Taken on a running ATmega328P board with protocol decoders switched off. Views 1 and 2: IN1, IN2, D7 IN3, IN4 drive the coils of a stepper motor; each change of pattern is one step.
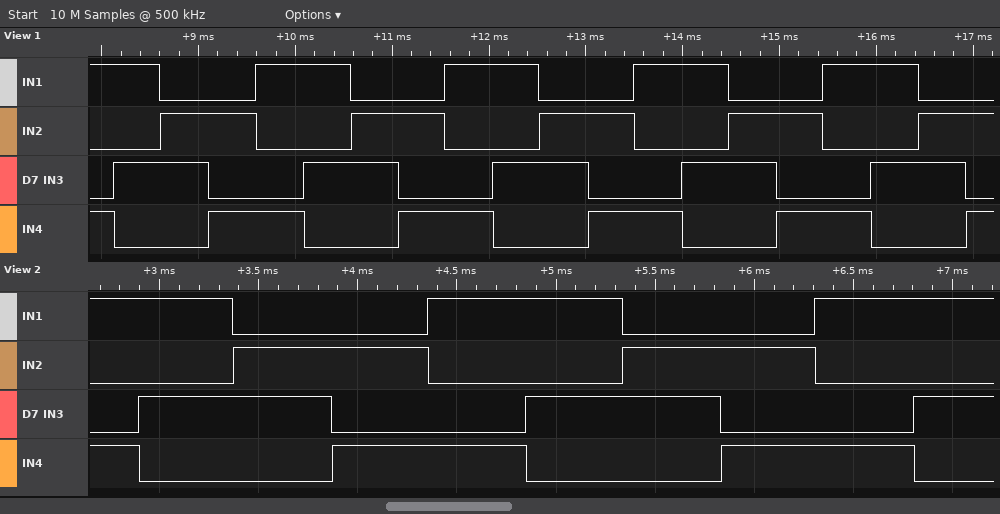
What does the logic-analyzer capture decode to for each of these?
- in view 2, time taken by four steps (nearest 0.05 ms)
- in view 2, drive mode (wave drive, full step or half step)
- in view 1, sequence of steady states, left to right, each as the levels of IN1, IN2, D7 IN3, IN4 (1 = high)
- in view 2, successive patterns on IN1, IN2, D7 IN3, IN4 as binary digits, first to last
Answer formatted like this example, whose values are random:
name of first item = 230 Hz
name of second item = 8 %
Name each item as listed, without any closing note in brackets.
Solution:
in view 2, time taken by four steps = 1.95 ms
in view 2, drive mode = full step
in view 1, sequence of steady states, left to right, each as the levels of IN1, IN2, D7 IN3, IN4 = 1001 1010 0110 0101 1001 1010 0110 0101 1001 1010 0110 0101 1001 1010 0110 0101 1001 1010 0110 0101
in view 2, successive patterns on IN1, IN2, D7 IN3, IN4 as binary digits, first to last = 1001 1010 0110 0101 1001 1010 0110 0101 1001 1010
